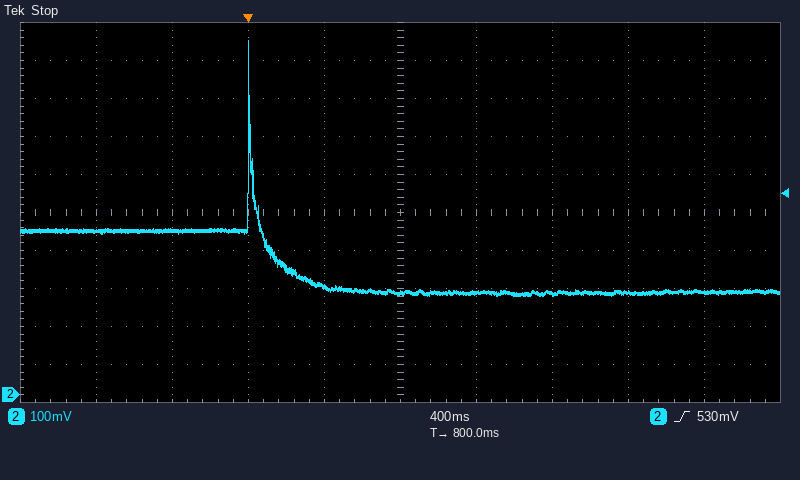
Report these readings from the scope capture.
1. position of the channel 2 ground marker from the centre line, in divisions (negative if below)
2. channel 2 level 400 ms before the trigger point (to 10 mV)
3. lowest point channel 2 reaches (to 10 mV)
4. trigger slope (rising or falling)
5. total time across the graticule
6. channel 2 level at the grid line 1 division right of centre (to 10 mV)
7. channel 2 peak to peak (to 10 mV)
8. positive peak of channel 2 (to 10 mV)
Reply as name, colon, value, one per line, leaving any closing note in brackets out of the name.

position of the channel 2 ground marker from the centre line, in divisions: -4.8 div
channel 2 level 400 ms before the trigger point: 430 mV
lowest point channel 2 reaches: 260 mV
trigger slope: rising
total time across the graticule: 4 s
channel 2 level at the grid line 1 division right of centre: 270 mV
channel 2 peak to peak: 670 mV
positive peak of channel 2: 930 mV
